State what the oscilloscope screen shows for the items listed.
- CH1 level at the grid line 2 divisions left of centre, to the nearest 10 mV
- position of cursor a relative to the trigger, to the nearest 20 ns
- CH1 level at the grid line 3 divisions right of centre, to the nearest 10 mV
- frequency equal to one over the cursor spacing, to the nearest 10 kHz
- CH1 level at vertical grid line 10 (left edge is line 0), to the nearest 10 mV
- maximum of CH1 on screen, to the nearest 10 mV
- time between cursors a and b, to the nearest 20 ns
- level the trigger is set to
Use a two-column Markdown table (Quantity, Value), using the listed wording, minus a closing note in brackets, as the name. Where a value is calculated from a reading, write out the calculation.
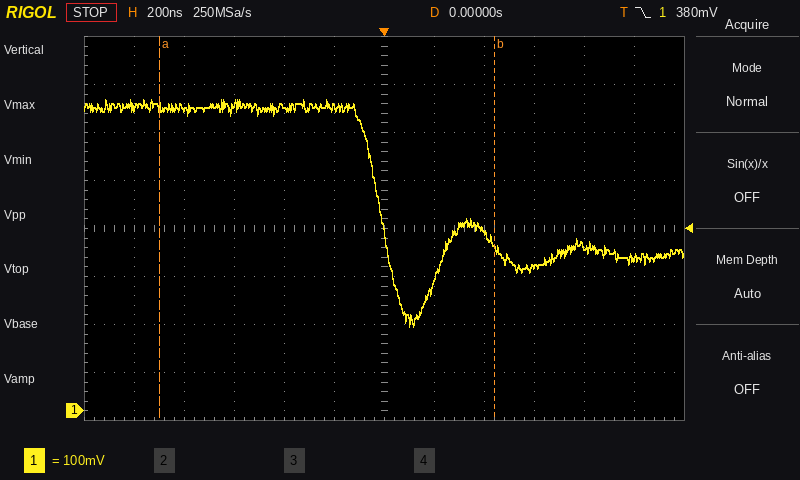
| Quantity | Value |
|---|---|
| CH1 level at the grid line 2 divisions left of centre, to the nearest 10 mV | 630 mV |
| position of cursor a relative to the trigger, to the nearest 20 ns | -900 ns |
| CH1 level at the grid line 3 divisions right of centre, to the nearest 10 mV | 300 mV |
| frequency equal to one over the cursor spacing, to the nearest 10 kHz | 1 / 1.34 µs ≈ 750 kHz |
| CH1 level at vertical grid line 10 (left edge is line 0), to the nearest 10 mV | 340 mV |
| maximum of CH1 on screen, to the nearest 10 mV | 650 mV |
| time between cursors a and b, to the nearest 20 ns | 1.34 µs |
| level the trigger is set to | 380 mV |
